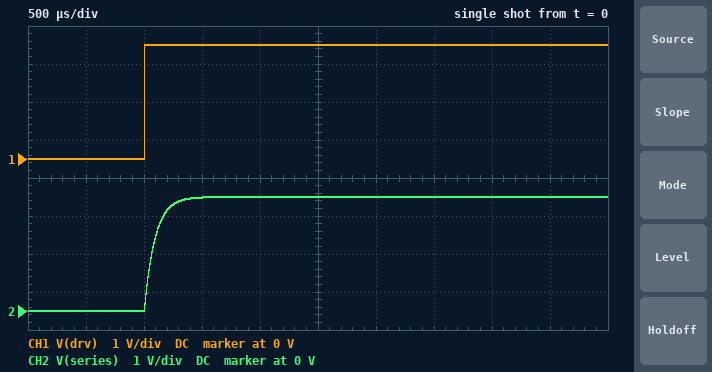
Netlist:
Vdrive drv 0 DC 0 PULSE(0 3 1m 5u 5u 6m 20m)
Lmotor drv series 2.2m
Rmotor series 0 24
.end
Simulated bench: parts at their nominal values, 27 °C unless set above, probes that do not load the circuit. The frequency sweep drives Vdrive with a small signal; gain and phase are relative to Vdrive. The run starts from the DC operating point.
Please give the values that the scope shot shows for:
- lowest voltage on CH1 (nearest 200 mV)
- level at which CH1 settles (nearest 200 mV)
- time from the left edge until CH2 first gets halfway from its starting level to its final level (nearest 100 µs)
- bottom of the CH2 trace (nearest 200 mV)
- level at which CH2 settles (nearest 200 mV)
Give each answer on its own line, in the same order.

0 V
3.0 V
1.1 ms
0 V
3.0 V
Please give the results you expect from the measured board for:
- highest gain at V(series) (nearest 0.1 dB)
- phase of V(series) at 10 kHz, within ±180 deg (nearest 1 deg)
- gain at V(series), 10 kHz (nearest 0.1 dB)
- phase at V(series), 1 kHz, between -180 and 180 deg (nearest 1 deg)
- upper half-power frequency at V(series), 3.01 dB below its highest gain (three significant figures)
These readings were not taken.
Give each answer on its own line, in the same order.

0 dB
-80 deg
-15.3 dB
-30 deg
1.74 kHz
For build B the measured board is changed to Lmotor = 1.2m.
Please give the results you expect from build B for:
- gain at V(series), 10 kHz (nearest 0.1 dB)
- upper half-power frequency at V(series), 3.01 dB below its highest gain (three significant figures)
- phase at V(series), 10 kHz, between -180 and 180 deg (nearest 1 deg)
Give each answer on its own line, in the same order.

-10.4 dB
3.18 kHz
-72 deg
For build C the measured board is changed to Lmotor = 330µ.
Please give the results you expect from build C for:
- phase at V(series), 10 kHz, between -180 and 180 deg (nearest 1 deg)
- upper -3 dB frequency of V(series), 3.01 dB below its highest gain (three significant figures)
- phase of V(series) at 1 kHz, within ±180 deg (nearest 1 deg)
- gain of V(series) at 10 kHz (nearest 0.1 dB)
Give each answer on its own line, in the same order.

-41 deg
11.6 kHz
-5 deg
-2.4 dB
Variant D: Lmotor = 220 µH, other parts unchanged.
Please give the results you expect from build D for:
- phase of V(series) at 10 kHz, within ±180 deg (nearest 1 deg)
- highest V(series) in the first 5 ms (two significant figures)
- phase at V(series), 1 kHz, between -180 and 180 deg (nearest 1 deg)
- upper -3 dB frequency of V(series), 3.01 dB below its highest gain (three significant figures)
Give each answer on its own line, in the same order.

-30 deg
3.0 V
-3 deg
17.4 kHz
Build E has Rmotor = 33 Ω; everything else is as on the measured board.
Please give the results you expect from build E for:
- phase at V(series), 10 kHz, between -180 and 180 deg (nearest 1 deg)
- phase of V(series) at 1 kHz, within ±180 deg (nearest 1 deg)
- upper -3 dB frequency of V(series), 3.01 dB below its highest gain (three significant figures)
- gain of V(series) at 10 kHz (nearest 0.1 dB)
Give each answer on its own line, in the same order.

-77 deg
-23 deg
2.39 kHz
-12.7 dB
